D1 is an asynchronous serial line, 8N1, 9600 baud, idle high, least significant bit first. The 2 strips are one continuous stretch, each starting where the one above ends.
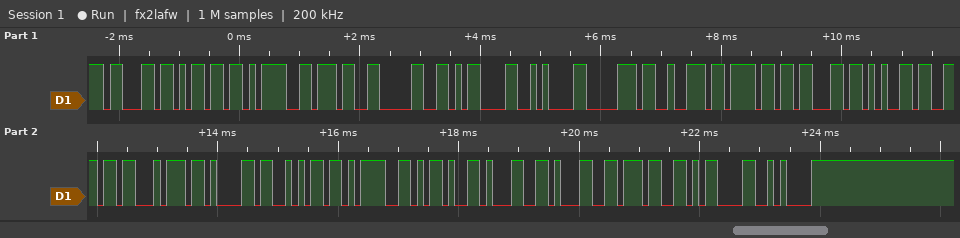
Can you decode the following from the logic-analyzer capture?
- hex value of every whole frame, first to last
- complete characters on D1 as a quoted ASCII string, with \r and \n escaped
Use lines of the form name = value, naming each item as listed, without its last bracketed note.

hex value of every whole frame, first to last = 63 6D 3D 37 30 0D 0A 70 72 6F 63 65 6E 74 61 6A 3D 2D 31 31 37 0D 0A
complete characters on D1 as a quoted ASCII string, with \r and \n escaped = "cm=70\r\nprocentaj=-117\r\n"
